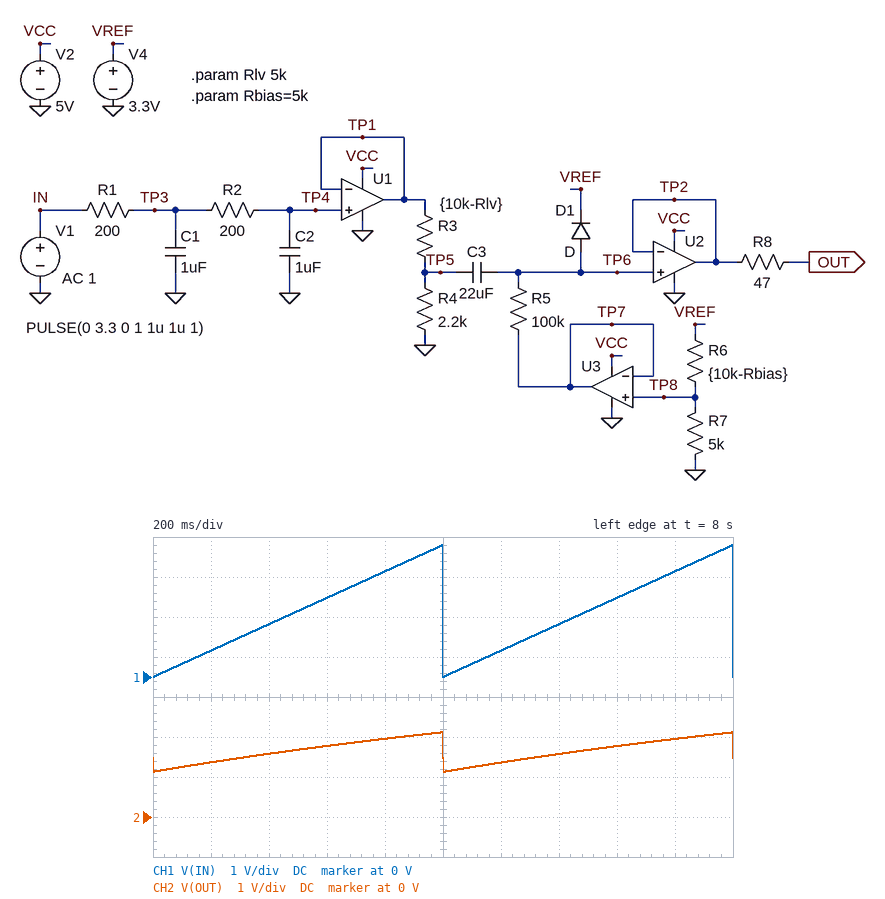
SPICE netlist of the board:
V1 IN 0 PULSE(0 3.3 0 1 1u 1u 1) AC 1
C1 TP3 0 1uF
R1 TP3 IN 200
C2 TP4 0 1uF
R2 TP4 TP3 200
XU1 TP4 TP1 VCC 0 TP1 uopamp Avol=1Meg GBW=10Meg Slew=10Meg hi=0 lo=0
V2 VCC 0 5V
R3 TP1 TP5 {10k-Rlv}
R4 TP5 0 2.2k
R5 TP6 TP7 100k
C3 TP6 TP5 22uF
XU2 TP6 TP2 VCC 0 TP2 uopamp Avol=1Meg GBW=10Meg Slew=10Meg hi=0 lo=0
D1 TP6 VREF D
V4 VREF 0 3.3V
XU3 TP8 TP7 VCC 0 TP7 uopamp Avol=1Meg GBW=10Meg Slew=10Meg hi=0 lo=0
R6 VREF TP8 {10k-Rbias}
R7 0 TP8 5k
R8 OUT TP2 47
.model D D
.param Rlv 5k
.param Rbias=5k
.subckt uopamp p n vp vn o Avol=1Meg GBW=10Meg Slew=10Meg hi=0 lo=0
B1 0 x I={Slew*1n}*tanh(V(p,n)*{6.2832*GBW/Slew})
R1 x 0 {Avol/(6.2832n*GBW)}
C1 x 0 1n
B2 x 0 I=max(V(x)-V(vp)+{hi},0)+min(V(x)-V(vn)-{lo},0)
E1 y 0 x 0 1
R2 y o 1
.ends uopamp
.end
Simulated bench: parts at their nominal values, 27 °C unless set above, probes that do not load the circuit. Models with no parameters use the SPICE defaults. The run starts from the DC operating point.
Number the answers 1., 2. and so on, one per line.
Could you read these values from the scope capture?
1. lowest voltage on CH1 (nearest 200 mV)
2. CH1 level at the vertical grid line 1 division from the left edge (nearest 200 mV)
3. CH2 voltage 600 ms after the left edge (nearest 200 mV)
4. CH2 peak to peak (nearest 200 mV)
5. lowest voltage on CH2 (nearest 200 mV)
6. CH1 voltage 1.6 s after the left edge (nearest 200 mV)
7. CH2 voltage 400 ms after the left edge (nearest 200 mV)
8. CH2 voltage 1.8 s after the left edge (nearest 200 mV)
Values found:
1. 0 V
2. 600 mV
3. 1.8 V
4. 1.0 V
5. 1.2 V
6. 2.0 V
7. 1.6 V
8. 2.0 V
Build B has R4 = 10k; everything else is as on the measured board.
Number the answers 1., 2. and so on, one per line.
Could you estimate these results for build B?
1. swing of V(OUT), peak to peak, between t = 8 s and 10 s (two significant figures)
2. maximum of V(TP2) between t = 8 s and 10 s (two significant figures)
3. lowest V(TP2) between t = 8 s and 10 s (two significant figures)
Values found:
1. 2.1 V
2. 2.7 V
3. 540 mV
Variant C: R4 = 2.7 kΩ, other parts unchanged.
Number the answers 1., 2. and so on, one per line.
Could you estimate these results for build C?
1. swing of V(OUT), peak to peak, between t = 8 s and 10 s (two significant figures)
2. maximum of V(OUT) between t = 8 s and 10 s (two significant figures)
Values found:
1. 1.1 V
2. 2.2 V
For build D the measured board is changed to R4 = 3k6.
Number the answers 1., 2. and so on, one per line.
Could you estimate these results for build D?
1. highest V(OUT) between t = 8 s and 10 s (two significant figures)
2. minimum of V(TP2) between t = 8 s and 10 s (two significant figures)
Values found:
1. 2.3 V
2. 940 mV
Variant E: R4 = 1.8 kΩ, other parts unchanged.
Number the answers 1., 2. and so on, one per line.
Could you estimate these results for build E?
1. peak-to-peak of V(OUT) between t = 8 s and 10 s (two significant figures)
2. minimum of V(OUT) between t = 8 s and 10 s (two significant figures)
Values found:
1. 860 mV
2. 1.2 V
